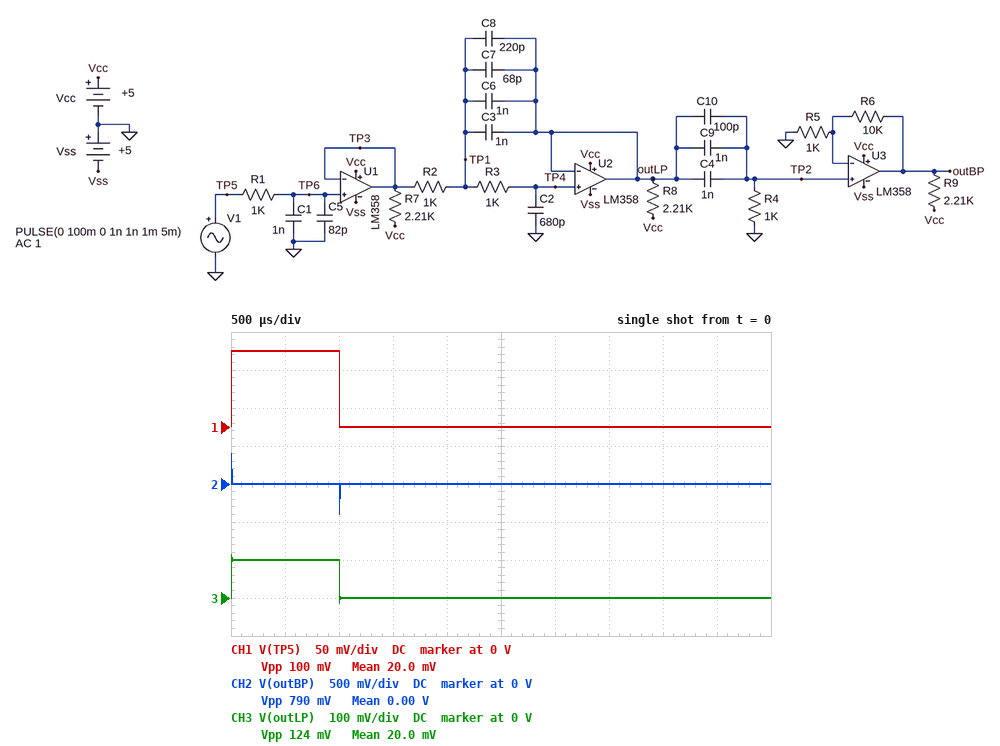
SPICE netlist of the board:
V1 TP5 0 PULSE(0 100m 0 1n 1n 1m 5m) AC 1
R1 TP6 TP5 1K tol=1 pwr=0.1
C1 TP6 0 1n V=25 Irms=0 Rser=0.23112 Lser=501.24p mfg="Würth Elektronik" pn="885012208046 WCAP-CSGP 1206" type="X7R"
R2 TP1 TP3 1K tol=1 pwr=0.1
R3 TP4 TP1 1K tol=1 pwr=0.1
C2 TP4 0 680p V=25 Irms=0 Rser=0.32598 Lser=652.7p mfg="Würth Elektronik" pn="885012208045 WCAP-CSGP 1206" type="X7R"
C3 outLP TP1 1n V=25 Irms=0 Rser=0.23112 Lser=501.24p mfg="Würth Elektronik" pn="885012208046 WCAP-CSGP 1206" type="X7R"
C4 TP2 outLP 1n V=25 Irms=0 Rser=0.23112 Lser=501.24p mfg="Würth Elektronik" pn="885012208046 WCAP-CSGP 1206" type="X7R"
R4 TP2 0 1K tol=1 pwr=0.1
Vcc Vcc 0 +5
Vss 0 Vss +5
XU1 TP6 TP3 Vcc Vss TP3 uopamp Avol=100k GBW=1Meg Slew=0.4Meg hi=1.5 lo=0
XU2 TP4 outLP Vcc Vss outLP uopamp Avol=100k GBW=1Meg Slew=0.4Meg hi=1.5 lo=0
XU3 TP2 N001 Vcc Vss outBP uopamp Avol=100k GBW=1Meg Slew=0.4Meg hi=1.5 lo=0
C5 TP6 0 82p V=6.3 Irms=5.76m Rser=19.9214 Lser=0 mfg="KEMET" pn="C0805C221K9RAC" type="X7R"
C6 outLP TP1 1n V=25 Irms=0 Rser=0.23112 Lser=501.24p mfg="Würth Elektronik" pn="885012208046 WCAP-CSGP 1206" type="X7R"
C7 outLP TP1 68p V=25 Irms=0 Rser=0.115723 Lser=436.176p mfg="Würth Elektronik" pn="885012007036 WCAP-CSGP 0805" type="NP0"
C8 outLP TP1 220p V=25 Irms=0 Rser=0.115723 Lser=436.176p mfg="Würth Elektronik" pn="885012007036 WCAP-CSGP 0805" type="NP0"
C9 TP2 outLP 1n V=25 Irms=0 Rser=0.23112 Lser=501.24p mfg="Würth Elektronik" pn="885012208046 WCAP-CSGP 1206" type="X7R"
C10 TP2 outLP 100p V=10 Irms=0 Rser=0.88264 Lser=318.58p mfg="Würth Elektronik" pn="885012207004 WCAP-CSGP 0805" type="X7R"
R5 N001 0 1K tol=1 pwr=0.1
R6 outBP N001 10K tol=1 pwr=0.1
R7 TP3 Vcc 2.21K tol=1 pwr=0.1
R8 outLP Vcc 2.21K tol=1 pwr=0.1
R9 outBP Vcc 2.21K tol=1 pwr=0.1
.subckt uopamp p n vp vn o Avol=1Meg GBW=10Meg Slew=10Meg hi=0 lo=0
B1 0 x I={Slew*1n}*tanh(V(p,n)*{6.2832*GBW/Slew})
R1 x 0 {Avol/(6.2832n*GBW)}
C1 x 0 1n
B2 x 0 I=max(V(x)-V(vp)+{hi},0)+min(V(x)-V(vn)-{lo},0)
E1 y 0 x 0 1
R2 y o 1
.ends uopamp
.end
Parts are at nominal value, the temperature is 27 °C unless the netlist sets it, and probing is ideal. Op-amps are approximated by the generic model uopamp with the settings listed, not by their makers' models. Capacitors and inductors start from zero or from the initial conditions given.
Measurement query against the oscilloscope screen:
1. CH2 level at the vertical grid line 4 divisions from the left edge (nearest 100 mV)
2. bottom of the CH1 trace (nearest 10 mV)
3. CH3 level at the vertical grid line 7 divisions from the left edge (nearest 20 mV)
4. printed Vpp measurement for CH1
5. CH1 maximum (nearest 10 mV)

0 V
0 V
0 V
100 mV
100 mV
